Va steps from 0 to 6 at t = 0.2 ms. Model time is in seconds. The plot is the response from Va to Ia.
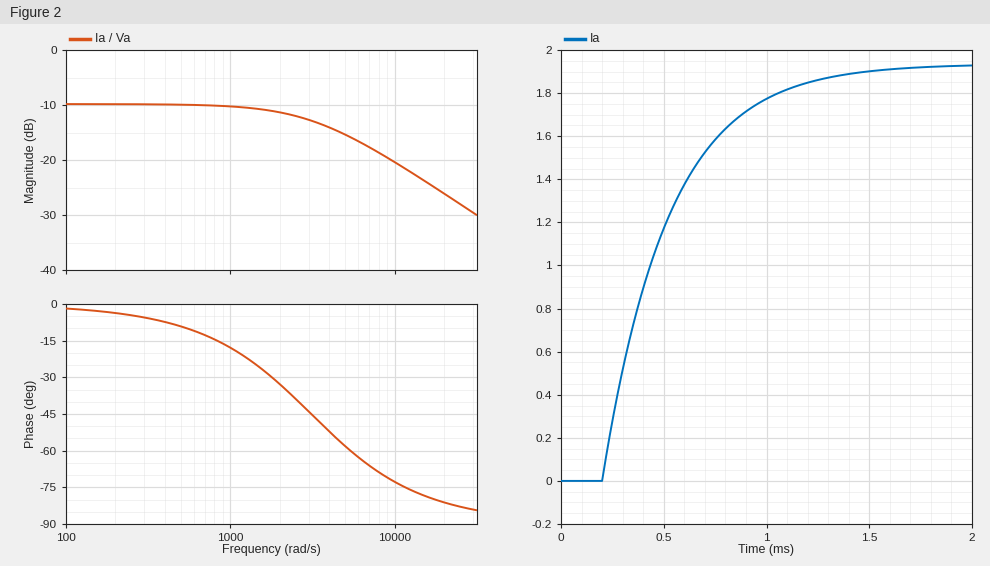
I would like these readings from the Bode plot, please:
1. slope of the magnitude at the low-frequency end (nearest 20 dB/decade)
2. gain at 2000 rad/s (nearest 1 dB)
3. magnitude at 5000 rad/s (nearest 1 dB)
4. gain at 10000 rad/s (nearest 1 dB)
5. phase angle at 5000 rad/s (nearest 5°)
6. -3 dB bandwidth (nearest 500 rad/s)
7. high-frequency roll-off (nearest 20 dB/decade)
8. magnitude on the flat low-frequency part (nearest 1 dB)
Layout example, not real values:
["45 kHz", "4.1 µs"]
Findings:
["0 dB/decade", "-11 dB", "-15 dB", "-20 dB", "-60°", "3000 rad/s", "-20 dB/decade", "-10 dB"]
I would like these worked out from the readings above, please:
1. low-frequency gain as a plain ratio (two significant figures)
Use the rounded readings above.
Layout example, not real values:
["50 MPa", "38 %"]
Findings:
["0.32"]
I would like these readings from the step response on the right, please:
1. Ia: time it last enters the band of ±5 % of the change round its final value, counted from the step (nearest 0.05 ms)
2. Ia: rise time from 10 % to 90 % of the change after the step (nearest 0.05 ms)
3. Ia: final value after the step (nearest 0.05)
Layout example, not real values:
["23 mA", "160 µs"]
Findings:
["0.95 ms", "0.70 ms", "1.95"]
